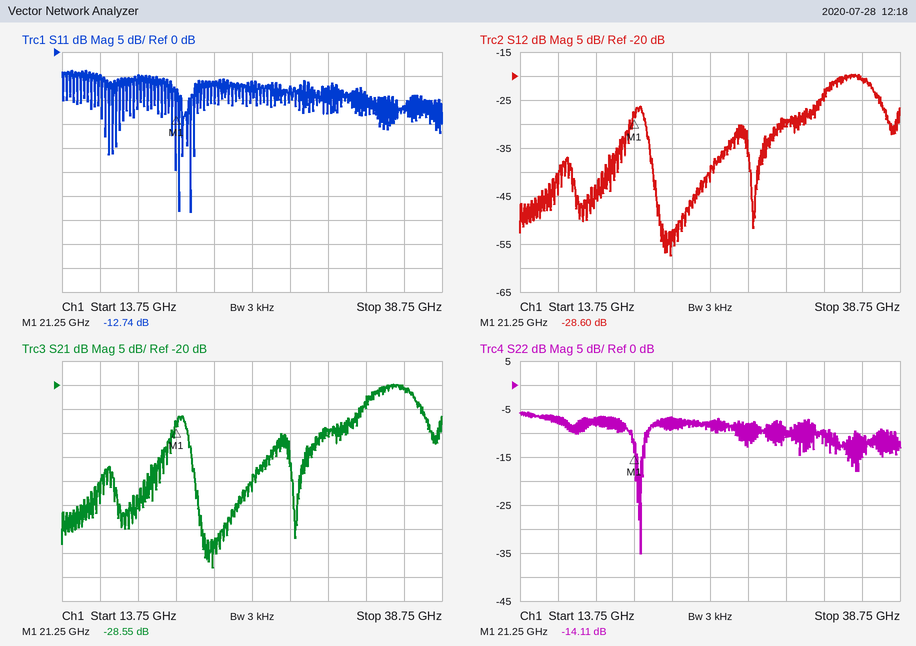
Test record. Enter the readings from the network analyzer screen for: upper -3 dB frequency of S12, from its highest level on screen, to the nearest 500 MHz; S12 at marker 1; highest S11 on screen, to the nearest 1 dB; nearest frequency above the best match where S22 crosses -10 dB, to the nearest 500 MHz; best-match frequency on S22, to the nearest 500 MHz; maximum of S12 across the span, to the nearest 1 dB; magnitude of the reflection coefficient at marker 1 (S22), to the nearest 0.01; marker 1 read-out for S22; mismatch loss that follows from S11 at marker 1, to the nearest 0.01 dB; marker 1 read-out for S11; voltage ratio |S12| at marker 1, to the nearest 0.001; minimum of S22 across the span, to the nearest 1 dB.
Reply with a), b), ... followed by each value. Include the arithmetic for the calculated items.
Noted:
a) 37.0 GHz
b) -28.60 dB
c) -4 dB
d) 22.0 GHz
e) 21.5 GHz
f) -20 dB
g) 10^(-14.11/20) ≈ 0.20
h) -14.11 dB
i) −10 log10(1 − 10^(-12.74/10)) ≈ 0.24 dB
j) -12.74 dB
k) 10^(-28.6/20) ≈ 0.037
l) -35 dB
